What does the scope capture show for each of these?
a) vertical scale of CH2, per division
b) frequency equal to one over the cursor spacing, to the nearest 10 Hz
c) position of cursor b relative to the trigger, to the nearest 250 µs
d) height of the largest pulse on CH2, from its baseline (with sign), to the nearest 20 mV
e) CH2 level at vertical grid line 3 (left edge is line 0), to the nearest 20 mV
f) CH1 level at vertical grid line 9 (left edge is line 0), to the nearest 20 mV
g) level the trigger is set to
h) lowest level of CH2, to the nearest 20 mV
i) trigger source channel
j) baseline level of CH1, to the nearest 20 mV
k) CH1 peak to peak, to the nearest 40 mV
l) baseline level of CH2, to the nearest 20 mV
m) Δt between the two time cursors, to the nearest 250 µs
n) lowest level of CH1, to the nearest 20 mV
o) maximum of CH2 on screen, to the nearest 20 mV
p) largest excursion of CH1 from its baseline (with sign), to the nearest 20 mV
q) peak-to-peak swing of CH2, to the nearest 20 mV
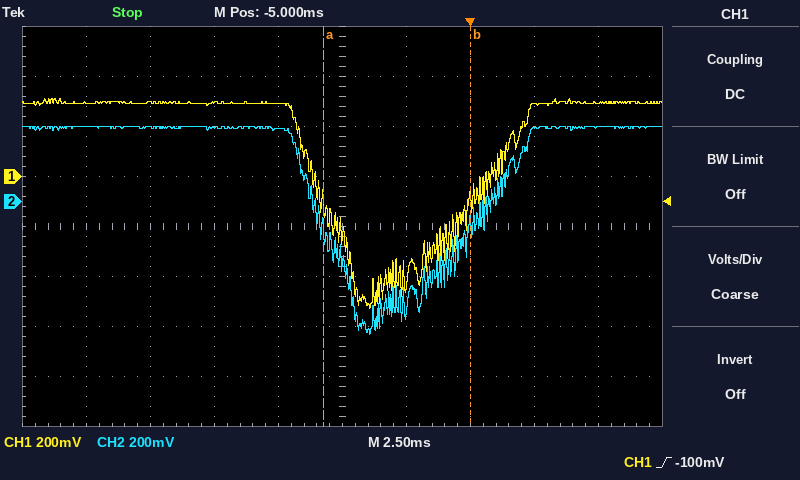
200 mV
170 Hz
0.00 ms
-840 mV
300 mV
300 mV
-100 mV
-540 mV
CH1
300 mV
840 mV
300 mV
5.75 ms
-520 mV
300 mV
-820 mV
840 mV
